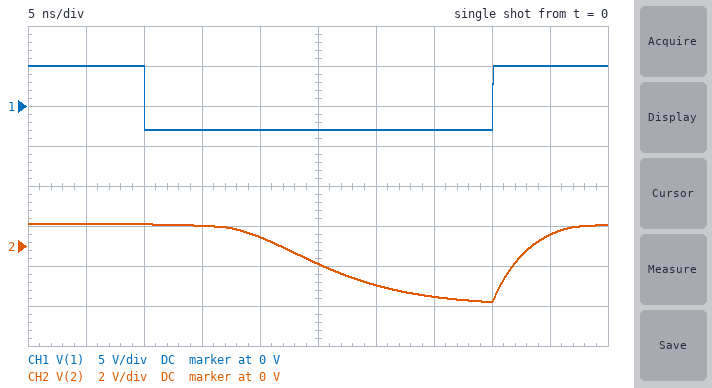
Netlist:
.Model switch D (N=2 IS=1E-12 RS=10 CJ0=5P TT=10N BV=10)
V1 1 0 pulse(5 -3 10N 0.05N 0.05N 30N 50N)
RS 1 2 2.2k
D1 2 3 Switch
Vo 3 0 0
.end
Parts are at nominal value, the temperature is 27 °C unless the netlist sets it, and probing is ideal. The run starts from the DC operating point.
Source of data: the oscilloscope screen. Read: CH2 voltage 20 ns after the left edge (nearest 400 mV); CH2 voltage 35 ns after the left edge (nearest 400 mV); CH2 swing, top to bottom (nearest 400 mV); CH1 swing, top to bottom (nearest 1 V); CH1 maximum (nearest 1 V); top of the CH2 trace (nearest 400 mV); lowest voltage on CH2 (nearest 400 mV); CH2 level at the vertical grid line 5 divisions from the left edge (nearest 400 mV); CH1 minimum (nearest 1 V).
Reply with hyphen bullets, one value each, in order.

- 400 mV
- -2.4 V
- 4.0 V
- 8 V
- 5 V
- 1.2 V
- -2.8 V
- -800 mV
- -3 V
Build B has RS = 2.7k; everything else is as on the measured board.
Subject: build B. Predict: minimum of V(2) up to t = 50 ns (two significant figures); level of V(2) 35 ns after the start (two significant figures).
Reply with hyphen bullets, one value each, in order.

- -2.6 V
- -2.2 V
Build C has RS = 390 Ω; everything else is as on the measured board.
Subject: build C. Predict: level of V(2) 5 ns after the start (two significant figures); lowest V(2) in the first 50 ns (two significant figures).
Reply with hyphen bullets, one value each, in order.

- 1.3 V
- -3.0 V
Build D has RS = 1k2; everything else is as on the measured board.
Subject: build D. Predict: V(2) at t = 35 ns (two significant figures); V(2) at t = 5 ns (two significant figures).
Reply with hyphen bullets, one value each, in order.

- -3.0 V
- 1.2 V
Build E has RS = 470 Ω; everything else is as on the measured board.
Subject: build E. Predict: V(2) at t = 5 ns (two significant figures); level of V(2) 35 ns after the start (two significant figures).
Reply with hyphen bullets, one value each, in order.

- 1.3 V
- -3.0 V
